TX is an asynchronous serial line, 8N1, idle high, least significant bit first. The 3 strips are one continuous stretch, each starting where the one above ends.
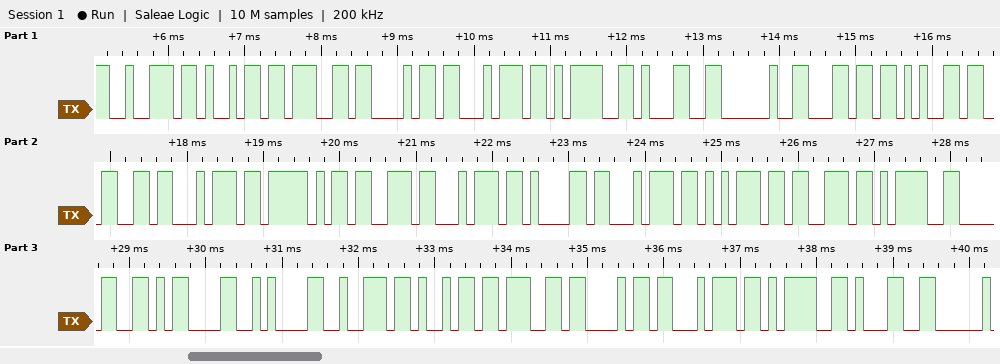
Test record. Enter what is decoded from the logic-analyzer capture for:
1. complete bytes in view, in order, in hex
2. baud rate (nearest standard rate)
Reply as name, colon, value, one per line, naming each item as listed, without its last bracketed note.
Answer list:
complete bytes in view, in order, in hex: 72 69 67 68 74 3D 31 20 6C 65 66 74 5F 73 74 61 74 75 73 3D 30 0D 0A 72 69 67 68 74 3D 31
baud rate: 9600 baud
